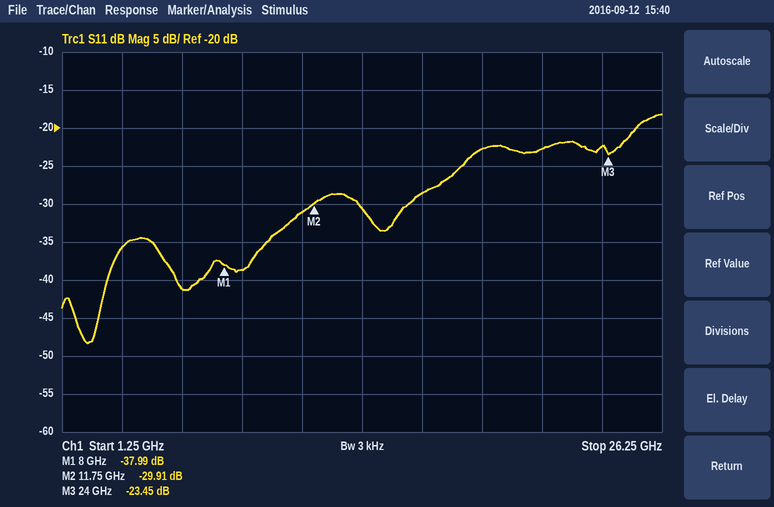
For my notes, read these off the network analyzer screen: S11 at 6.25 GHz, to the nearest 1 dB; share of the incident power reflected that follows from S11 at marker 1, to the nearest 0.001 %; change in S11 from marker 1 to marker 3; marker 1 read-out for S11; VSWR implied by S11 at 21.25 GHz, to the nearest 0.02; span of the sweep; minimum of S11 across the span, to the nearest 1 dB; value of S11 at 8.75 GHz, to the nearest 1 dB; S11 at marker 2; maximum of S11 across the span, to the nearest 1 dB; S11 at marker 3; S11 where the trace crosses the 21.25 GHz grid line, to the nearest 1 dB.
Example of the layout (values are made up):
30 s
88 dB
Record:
-41 dB
0.016 %
14.54 dB
-37.99 dB
1.16
25 GHz
-48 dB
-39 dB
-29.91 dB
-18 dB
-23.45 dB
-23 dB
